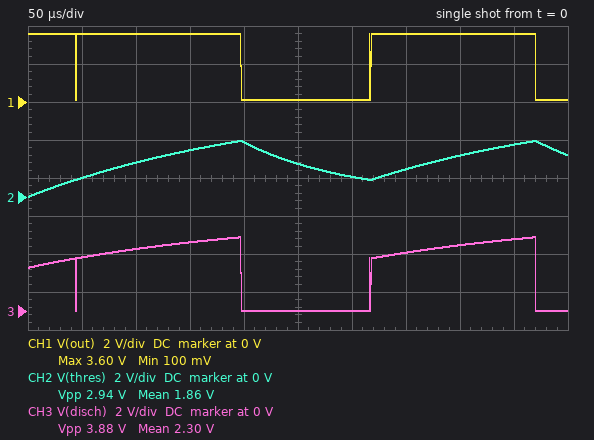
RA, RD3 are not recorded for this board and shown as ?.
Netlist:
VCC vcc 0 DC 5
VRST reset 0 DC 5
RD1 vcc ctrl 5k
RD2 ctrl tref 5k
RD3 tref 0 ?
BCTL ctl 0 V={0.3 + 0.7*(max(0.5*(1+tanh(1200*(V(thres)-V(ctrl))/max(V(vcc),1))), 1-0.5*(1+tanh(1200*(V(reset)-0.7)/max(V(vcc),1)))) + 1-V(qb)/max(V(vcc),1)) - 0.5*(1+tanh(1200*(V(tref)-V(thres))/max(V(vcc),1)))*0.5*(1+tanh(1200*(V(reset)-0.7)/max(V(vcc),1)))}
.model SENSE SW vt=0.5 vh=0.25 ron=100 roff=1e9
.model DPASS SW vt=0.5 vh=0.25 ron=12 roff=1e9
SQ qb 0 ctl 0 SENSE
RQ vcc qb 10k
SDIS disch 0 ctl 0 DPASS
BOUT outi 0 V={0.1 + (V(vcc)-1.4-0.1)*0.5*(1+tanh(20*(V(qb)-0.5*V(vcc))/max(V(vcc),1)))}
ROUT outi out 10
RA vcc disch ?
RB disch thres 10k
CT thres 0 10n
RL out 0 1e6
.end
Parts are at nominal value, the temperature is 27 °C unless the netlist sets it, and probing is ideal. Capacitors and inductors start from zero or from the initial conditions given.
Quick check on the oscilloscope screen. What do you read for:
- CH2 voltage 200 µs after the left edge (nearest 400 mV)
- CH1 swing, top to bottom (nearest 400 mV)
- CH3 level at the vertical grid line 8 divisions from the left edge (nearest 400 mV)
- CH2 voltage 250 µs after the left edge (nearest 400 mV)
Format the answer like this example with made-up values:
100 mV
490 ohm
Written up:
2.8 V
3.6 V
3.6 V
1.6 V
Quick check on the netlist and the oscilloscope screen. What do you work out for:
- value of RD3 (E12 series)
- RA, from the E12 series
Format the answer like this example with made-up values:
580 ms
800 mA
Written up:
2.2 kΩ
12 kΩ
